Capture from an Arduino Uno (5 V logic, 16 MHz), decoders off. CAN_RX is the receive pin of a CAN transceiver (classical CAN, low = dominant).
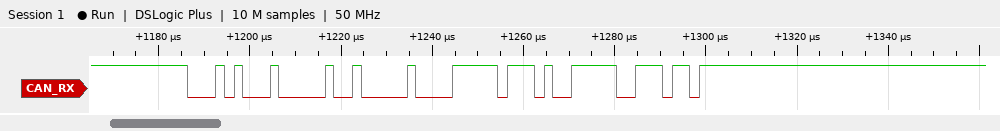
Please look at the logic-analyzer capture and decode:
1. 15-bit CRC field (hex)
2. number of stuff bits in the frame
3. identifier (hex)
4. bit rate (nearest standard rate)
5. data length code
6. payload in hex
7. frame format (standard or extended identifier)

0x27DD
4
0x144
500 kbit/s
2
00 FF
standard
